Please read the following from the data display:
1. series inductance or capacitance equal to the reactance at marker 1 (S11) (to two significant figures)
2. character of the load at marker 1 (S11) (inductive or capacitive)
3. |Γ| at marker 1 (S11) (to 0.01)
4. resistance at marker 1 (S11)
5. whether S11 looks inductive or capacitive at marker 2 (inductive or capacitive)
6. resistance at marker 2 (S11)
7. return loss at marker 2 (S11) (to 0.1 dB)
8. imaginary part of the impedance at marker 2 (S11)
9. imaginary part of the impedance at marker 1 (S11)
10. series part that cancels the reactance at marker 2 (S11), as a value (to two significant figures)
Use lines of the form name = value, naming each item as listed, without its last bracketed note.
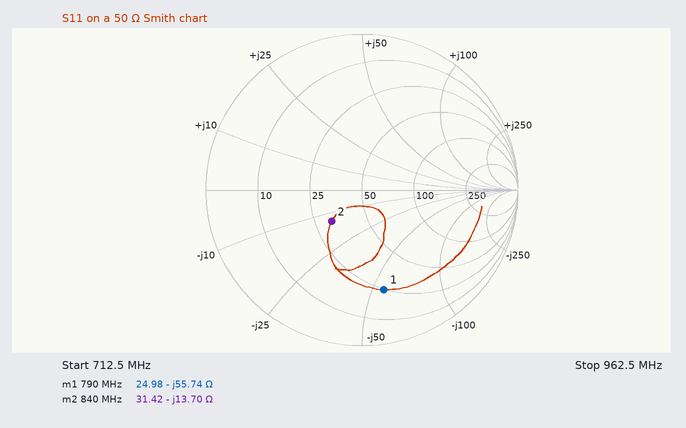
series inductance or capacitance equal to the reactance at marker 1 (S11) = 3.6 pF
character of the load at marker 1 (S11) = capacitive
|Γ| at marker 1 (S11) = 0.65
resistance at marker 1 = 24.98 Ω
whether S11 looks inductive or capacitive at marker 2 = capacitive
resistance at marker 2 = 31.42 Ω
return loss at marker 2 (S11) = 11.1 dB
imaginary part of the impedance at marker 2 = -13.70 Ω
imaginary part of the impedance at marker 1 = -55.74 Ω
series part that cancels the reactance at marker 2 (S11), as a value = 2.6 nH
